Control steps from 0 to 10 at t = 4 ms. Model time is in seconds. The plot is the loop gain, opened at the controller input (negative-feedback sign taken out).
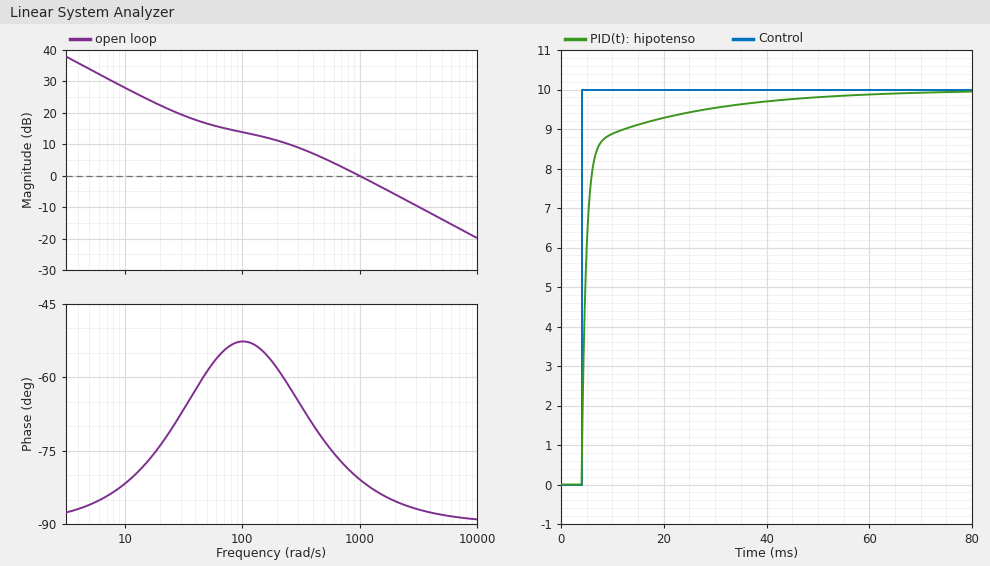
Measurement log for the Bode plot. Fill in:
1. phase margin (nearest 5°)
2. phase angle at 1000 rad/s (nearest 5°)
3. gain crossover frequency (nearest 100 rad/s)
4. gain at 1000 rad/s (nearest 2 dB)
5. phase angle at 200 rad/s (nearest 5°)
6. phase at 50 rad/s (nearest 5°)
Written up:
100°
-80°
1000 rad/s
0 dB
-60°
-60°
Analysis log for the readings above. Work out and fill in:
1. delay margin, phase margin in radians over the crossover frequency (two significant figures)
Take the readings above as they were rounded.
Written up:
0.0017 s
